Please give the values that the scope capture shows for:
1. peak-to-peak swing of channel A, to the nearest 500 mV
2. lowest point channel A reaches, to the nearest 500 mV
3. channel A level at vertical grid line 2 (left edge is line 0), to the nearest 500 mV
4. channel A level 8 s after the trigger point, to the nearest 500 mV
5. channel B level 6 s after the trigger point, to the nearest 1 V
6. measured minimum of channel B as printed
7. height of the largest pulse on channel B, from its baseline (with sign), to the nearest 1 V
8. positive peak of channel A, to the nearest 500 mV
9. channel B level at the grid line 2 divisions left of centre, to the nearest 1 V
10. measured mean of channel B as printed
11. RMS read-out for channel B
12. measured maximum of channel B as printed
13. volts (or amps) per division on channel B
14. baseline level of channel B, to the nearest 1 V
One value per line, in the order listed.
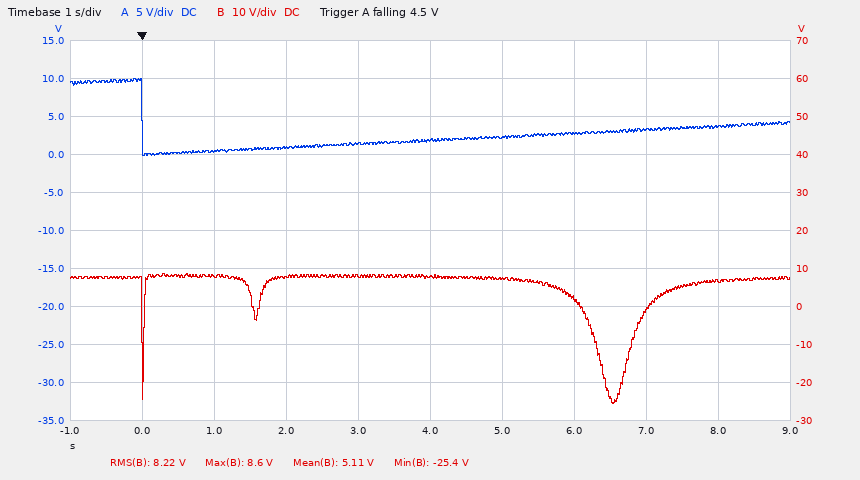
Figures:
10.0 V
0.0 V
500 mV
3.5 V
2 V
-25.4 V
-33 V
10.0 V
8 V
5.11 V
8.22 V
8.6 V
10 V
8 V
